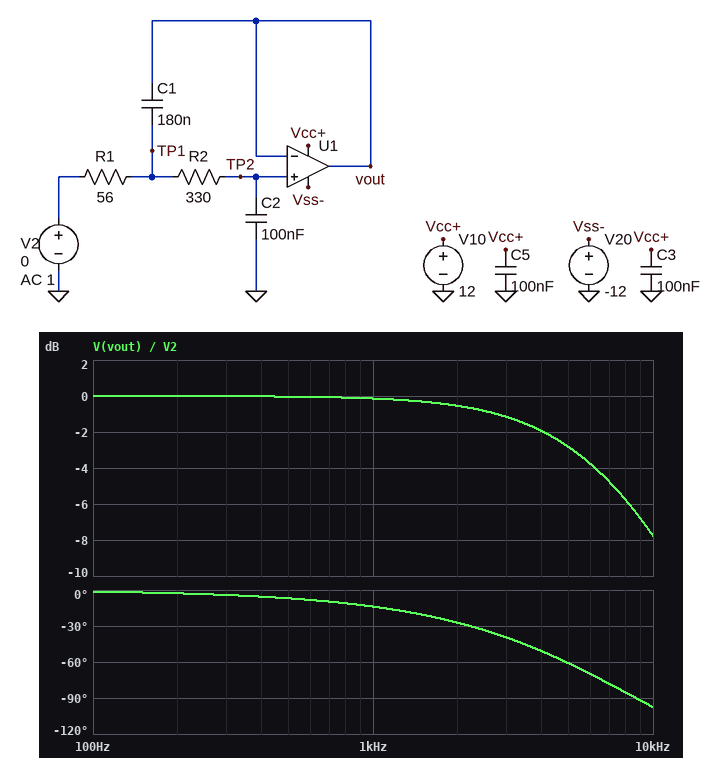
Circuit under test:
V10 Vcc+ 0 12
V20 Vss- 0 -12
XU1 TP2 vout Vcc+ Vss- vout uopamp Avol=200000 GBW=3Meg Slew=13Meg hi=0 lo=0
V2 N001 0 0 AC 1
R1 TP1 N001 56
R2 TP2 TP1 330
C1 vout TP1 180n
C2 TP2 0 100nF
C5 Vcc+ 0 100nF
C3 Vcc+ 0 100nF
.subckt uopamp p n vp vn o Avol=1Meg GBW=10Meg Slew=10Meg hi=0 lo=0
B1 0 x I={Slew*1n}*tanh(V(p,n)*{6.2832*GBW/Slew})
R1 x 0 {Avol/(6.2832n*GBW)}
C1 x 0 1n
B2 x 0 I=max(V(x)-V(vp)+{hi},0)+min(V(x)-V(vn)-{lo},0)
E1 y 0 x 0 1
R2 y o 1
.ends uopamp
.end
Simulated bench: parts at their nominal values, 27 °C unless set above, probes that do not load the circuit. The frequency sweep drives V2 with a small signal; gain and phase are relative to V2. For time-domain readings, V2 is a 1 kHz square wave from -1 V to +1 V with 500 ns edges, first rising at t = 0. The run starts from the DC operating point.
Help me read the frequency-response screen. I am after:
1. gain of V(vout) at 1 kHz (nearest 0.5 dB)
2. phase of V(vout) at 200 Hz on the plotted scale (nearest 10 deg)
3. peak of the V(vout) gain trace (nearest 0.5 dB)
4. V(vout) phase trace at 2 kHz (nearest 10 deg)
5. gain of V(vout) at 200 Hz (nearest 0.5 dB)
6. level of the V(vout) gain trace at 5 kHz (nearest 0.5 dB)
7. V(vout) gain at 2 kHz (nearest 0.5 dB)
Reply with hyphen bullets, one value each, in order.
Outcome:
- 0 dB
- 0 deg
- 0 dB
- -30 deg
- 0 dB
- -3.0 dB
- -0.5 dB
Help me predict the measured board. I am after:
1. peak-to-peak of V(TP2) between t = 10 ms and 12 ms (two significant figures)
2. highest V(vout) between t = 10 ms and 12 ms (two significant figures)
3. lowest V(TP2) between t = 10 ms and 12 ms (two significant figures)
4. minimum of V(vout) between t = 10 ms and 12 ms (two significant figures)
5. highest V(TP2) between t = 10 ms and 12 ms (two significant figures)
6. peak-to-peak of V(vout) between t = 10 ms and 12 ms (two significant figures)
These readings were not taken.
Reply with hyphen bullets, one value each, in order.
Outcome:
- 2.0 V
- 1.0 V
- -1.0 V
- -1.0 V
- 1.0 V
- 2.0 V
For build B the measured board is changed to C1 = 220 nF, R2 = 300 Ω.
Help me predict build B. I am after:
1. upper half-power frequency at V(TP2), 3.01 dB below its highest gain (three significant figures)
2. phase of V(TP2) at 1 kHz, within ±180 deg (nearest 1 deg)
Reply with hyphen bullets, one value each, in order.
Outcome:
- 5.94 kHz
- -13 deg
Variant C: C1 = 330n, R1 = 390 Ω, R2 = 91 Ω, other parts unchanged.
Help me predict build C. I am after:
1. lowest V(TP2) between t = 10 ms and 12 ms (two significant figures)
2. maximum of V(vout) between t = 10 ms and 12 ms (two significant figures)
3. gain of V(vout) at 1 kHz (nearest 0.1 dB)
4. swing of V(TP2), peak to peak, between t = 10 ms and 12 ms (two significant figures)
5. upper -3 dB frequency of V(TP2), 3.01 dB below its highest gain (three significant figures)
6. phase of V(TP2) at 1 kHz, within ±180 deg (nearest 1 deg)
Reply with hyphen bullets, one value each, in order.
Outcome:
- -1.1 V
- 1.1 V
- 0 dB
- 2.2 V
- 4.68 kHz
- -18 deg
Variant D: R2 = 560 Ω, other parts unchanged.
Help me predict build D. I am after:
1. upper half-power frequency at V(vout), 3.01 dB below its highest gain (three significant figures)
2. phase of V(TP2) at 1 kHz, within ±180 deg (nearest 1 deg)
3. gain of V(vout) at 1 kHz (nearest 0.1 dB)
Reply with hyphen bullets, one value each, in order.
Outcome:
- 3.02 kHz
- -22 deg
- -0.4 dB
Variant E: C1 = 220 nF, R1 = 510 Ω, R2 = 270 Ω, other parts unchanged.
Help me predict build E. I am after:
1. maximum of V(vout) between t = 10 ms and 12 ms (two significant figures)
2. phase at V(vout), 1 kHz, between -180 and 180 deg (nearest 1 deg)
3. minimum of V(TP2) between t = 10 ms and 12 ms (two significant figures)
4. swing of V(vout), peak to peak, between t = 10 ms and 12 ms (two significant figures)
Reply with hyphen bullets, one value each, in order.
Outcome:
- 1.1 V
- -29 deg
- -1.1 V
- 2.2 V
